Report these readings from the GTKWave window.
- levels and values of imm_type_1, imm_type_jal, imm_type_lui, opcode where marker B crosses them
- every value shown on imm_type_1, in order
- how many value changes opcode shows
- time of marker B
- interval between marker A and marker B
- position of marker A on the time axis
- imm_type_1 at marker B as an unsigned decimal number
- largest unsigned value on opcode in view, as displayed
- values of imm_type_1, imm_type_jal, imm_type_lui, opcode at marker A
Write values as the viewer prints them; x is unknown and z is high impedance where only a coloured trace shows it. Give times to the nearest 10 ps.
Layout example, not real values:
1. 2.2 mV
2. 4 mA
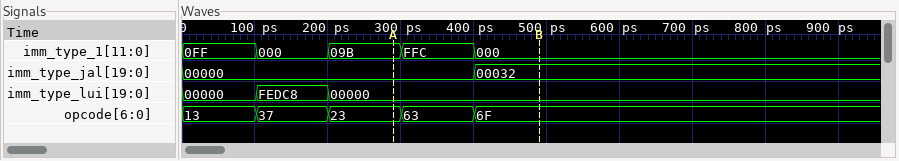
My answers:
1. imm_type_1=000, imm_type_jal=00032, imm_type_lui=00000, opcode=6F
2. 0FF, 000, 09B, FFC, 000
3. 4
4. 490 ps
5. 200 ps
6. 290 ps
7. 0
8. 6F
9. imm_type_1=09B, imm_type_jal=00000, imm_type_lui=00000, opcode=23
